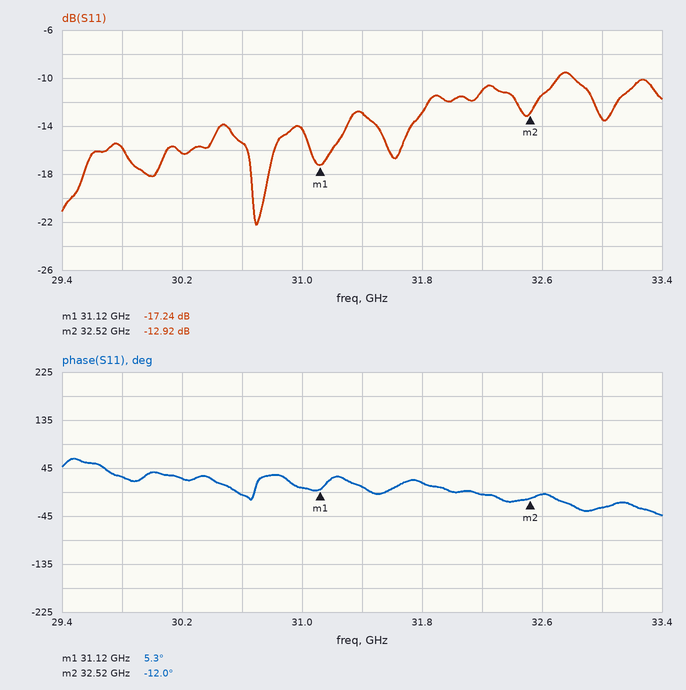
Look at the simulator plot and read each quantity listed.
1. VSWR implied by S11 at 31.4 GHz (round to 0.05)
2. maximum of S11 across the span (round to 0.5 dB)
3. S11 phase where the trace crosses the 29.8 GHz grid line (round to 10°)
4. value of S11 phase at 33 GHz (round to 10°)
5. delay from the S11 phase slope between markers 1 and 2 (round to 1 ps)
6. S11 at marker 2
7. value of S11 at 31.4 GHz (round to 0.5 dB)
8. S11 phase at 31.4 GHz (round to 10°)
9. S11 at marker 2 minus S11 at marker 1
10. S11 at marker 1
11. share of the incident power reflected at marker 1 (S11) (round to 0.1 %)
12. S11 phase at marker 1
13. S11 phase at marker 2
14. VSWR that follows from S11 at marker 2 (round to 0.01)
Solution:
1.60
-9.5 dB
30°
-30°
34 ps
-12.92 dB
-13.0 dB
10°
4.32 dB
-17.24 dB
1.9 %
5.3°
-12.0°
1.58
